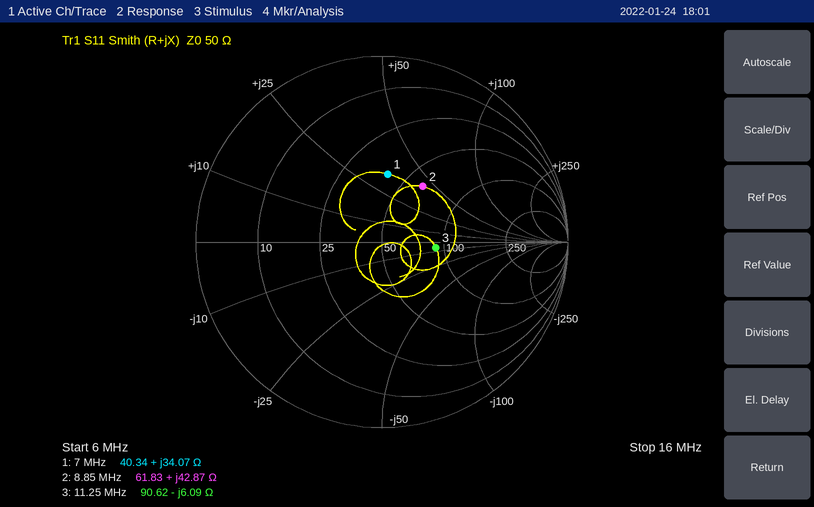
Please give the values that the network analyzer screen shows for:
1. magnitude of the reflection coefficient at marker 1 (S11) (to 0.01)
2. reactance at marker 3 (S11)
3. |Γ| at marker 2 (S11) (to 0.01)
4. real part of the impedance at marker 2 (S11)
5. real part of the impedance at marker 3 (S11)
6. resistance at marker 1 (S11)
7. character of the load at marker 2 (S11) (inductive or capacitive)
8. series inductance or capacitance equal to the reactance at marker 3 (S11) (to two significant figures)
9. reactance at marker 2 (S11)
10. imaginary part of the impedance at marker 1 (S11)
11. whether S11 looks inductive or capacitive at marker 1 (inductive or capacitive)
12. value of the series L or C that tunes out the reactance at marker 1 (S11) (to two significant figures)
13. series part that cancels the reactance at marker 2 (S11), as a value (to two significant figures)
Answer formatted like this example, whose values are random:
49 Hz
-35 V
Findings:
0.37
-6.09 Ω
0.37
61.83 Ω
90.62 Ω
40.34 Ω
inductive
2.3 nF
+42.87 Ω
+34.07 Ω
inductive
670 pF
420 pF
